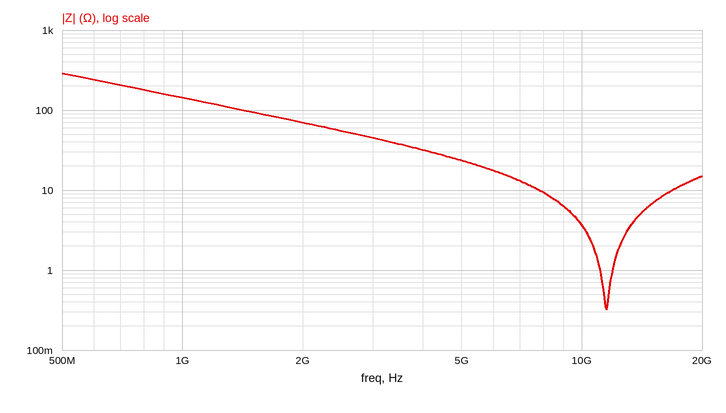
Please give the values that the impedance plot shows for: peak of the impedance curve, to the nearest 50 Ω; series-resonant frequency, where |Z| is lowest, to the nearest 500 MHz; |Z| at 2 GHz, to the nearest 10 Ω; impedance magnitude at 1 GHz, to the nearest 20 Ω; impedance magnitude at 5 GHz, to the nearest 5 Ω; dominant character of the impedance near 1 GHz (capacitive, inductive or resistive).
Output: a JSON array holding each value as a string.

["300 Ω", "11.5 GHz", "70 Ω", "140 Ω", "25 Ω", "capacitive"]
